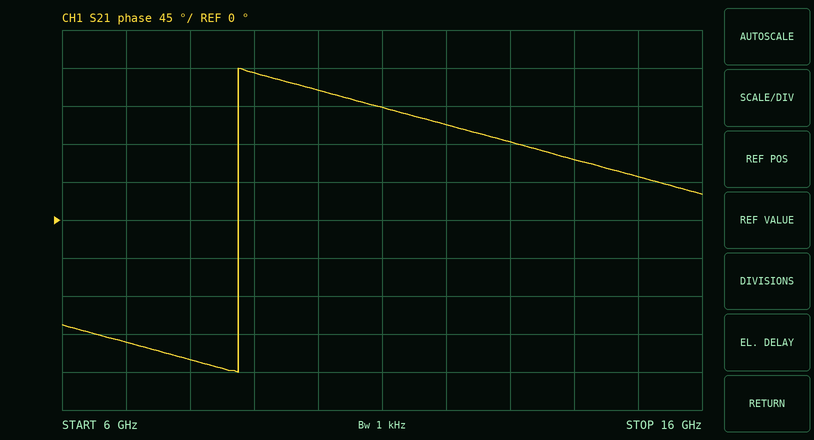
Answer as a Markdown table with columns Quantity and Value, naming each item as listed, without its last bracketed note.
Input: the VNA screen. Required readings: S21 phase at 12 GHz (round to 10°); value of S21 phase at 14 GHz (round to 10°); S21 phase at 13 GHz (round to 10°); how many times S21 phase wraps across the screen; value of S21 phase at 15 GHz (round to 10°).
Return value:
| Quantity | Value |
|---|---|
| S21 phase at 12 GHz | 110° |
| value of S21 phase at 14 GHz | 70° |
| S21 phase at 13 GHz | 90° |
| how many times S21 phase wraps across the screen | 1 |
| value of S21 phase at 15 GHz | 50° |
